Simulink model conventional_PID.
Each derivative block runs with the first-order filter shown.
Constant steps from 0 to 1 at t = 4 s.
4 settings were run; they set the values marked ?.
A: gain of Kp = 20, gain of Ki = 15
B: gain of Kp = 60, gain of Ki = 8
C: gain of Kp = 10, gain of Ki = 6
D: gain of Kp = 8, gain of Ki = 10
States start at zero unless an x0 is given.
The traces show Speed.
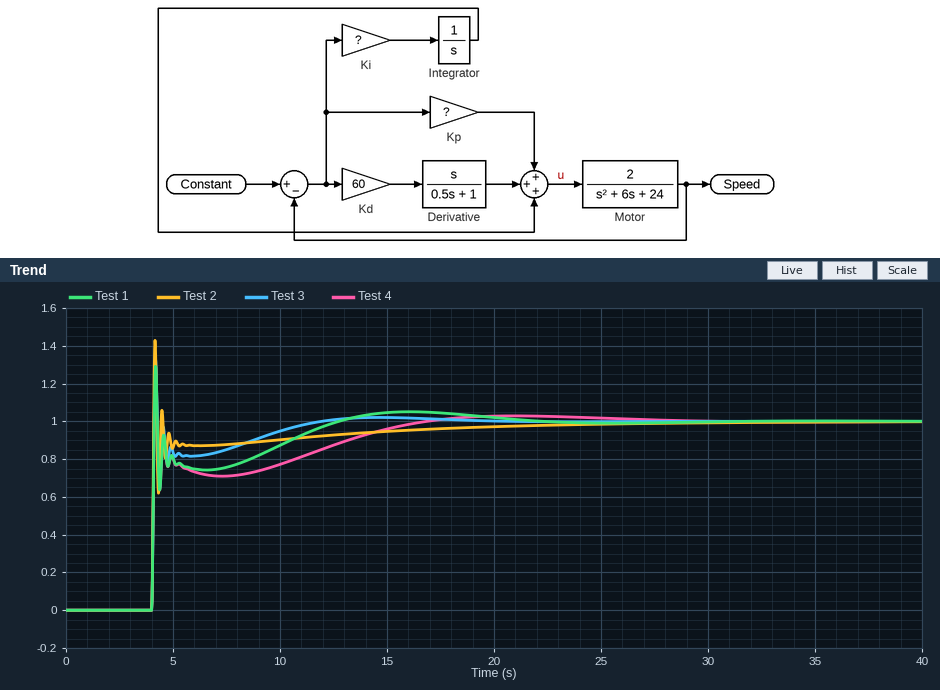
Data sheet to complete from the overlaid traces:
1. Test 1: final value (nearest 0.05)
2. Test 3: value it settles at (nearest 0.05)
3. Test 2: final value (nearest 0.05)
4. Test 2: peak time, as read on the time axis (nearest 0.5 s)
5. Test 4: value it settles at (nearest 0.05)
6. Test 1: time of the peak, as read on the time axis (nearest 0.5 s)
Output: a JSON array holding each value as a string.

["1.00", "1.00", "1.00", "4.0 s", "1.00", "4.0 s"]
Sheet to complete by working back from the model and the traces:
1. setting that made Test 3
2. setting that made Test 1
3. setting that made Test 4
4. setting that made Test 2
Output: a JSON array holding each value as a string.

["A", "D", "C", "B"]
